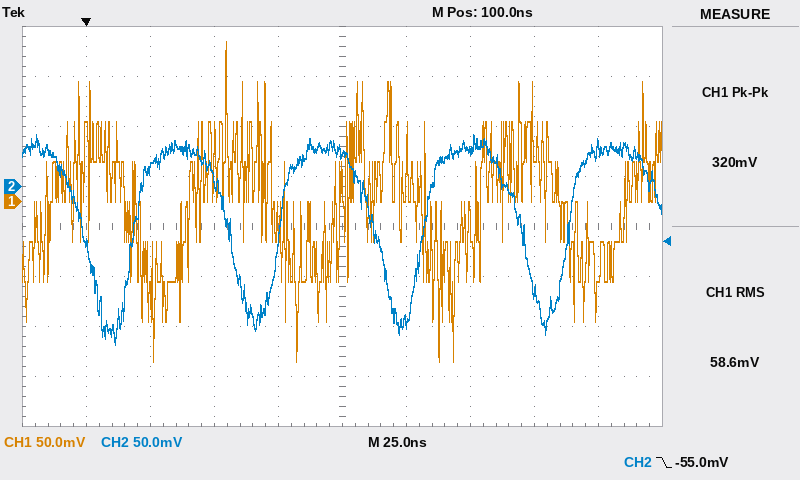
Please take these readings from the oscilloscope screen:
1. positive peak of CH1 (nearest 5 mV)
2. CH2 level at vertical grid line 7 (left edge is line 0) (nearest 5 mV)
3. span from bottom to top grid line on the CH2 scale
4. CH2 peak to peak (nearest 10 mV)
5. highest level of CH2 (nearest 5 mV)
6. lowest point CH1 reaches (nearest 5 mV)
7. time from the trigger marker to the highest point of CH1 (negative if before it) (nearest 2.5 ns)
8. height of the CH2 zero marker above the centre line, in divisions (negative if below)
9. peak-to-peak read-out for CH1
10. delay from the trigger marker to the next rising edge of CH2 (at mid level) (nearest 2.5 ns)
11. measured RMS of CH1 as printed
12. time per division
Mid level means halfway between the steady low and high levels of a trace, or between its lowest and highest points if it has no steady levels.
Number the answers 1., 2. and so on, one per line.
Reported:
1. 160 mV
2. 35 mV
3. 400 mV
4. 210 mV
5. 50 mV
6. -160 mV
7. +55.0 ns
8. +0.8 div
9. 320 mV
10. 17.5 ns
11. 58.6 mV
12. 25 ns
